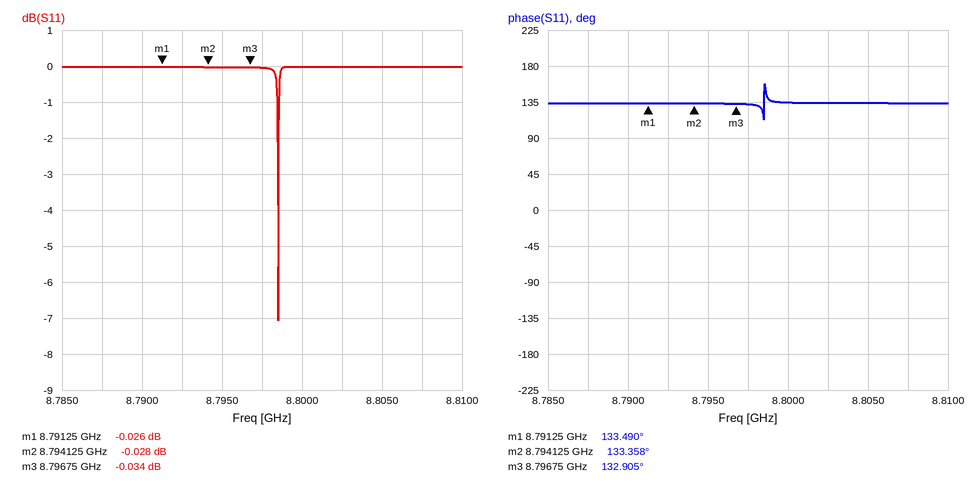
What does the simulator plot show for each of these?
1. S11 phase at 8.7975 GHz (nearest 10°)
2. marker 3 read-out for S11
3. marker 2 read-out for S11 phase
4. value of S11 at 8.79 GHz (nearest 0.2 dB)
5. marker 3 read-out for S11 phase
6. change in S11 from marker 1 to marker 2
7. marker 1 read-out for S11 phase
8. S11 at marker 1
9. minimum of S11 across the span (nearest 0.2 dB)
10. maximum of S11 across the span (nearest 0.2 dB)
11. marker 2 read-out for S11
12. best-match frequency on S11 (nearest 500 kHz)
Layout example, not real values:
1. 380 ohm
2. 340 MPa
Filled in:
1. 130°
2. -0.034 dB
3. 133.358°
4. 0.0 dB
5. 132.905°
6. -0.002 dB
7. 133.490°
8. -0.026 dB
9. -7.0 dB
10. 0.0 dB
11. -0.028 dB
12. 8.7985 GHz
